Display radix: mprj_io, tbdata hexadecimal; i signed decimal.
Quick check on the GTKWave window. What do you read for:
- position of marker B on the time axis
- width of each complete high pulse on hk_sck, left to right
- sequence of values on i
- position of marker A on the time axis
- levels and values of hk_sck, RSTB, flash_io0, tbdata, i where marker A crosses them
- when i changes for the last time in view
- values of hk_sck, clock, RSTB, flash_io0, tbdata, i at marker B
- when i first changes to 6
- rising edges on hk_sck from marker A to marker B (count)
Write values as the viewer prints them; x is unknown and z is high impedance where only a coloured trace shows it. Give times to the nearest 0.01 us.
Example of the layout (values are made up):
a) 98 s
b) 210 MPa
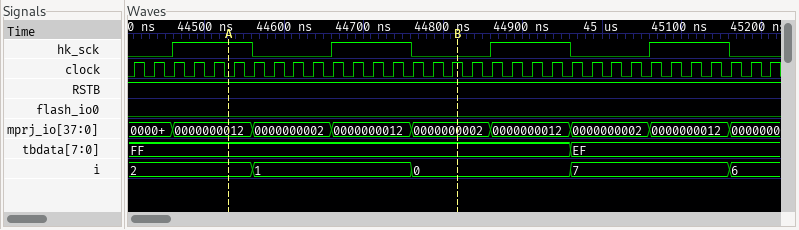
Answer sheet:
a) 44.82 us
b) 0.1 us, 0.1 us, 0.1 us, 0.1 us
c) 2, 1, 0, 7, 6
d) 44.53 us
e) hk_sck=1, RSTB=1, flash_io0=0, tbdata=FF, i=2
f) 45.16 us
g) hk_sck=0, clock=1, RSTB=1, flash_io0=0, tbdata=FF, i=0
h) 45.16 us
i) 1
